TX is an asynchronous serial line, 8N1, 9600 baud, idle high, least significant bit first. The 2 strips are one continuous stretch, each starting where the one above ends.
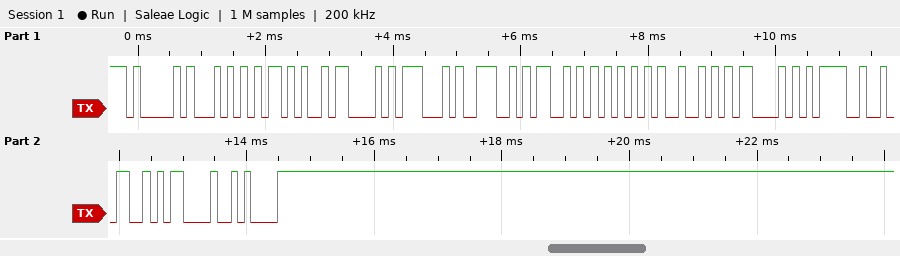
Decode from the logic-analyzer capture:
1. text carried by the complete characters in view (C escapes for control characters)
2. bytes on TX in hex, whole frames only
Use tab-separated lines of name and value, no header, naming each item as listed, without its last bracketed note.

text carried by the complete characters in view	"AT+CGNSURC=2\r\n"
bytes on TX in hex, whole frames only	41 54 2B 43 47 4E 53 55 52 43 3D 32 0D 0A
